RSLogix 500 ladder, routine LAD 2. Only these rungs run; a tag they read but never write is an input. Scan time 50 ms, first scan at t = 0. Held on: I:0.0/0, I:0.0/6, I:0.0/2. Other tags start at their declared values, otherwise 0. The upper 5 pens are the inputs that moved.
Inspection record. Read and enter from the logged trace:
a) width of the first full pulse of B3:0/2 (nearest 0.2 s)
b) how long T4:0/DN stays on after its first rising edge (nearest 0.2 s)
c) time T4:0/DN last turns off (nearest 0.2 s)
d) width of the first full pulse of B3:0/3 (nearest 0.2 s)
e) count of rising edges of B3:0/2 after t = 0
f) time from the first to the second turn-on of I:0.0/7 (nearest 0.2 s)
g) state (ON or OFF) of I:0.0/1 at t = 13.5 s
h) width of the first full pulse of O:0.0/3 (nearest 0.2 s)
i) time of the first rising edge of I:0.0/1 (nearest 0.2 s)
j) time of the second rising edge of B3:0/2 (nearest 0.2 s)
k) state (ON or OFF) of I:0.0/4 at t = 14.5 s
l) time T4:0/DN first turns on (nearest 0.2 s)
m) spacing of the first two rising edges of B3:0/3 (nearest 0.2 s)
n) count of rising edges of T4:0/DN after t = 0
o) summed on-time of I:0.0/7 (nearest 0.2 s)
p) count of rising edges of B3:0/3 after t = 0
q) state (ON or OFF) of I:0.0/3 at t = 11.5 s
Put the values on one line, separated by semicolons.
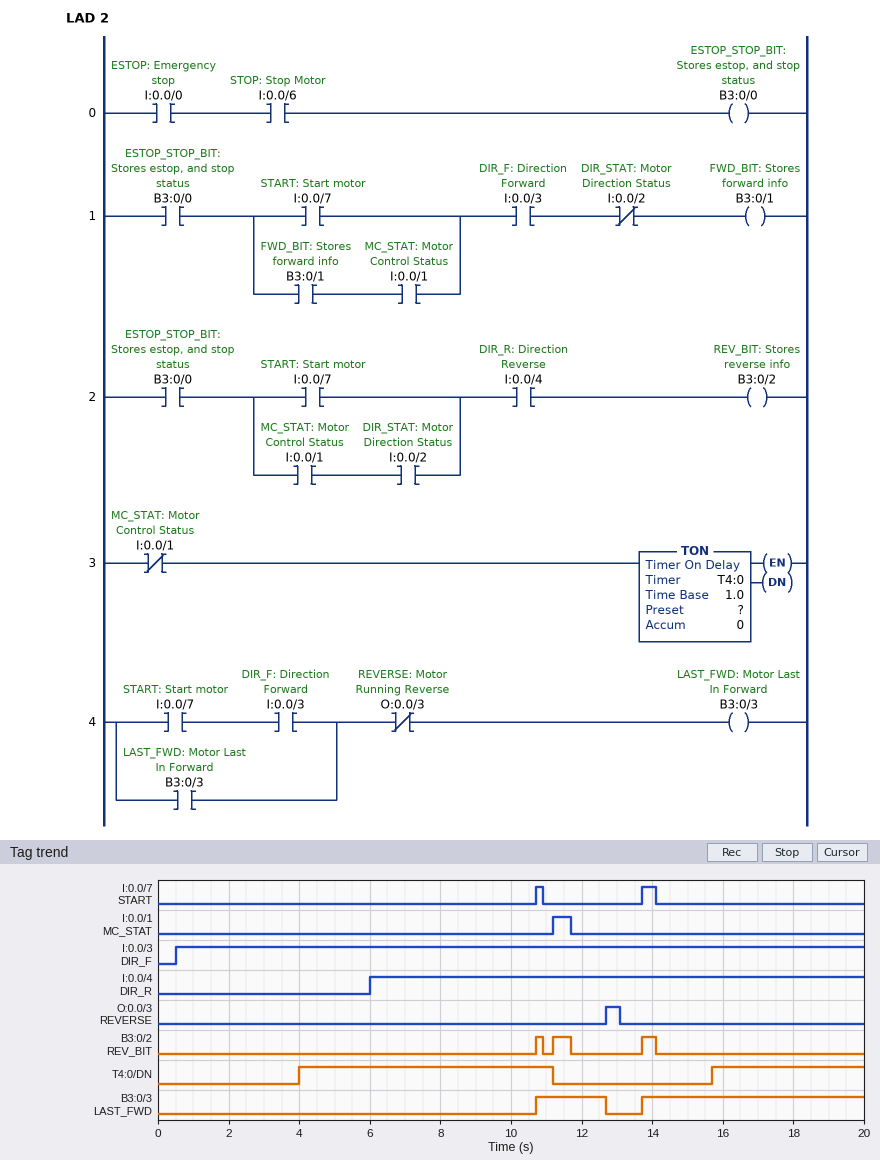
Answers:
0.2 s; 7.2 s; 11.2 s; 2.0 s; 3; 3.0 s; OFF; 0.4 s; 11.2 s; 11.2 s; ON; 4.0 s; 3.0 s; 2; 0.6 s; 2; ON
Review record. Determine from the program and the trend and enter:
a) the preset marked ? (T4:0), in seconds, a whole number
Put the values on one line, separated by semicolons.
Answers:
4 s
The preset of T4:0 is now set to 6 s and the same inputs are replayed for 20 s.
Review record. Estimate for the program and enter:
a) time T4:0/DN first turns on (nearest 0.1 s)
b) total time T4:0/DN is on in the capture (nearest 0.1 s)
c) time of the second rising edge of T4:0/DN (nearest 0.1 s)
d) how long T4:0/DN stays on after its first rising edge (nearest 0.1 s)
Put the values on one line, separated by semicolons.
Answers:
6.0 s; 7.5 s; 17.7 s; 5.2 s
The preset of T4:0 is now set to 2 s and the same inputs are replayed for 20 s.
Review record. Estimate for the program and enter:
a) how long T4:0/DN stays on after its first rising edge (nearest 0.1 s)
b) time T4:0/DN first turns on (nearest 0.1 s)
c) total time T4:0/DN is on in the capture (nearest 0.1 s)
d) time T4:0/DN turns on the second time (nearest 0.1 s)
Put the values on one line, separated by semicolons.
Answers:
9.2 s; 2.0 s; 15.5 s; 13.7 s
